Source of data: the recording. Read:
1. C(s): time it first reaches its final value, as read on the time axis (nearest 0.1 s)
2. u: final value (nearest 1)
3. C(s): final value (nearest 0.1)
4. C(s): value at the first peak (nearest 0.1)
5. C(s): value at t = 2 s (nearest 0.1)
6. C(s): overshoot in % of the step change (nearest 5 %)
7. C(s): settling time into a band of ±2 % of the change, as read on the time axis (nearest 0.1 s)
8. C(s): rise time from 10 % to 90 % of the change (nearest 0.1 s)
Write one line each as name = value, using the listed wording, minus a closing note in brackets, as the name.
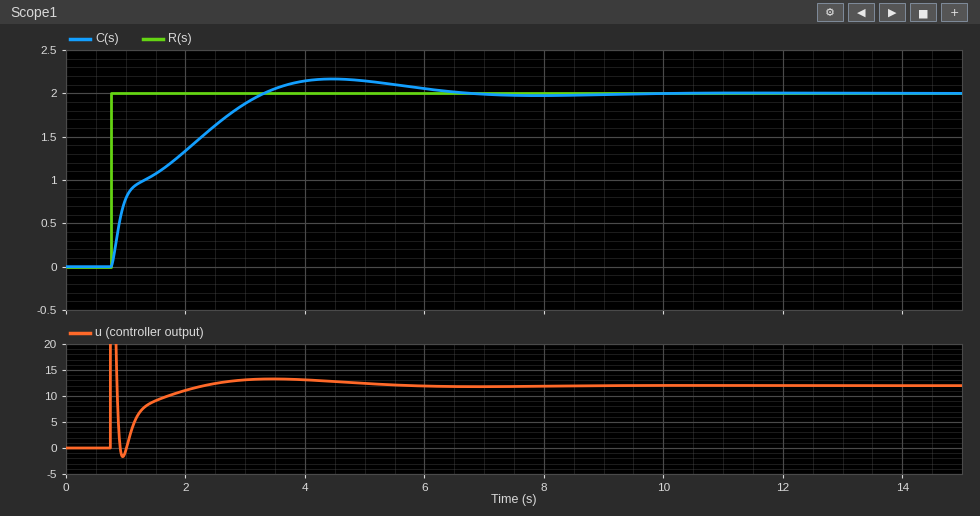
C(s): time it first reaches its final value, as read on the time axis = 3.3 s
u: final value = 12
C(s): final value = 2.0
C(s): value at the first peak = 2.2
C(s): value at t = 2 s = 1.3
C(s): overshoot in % of the step change = 10 %
C(s): settling time into a band of ±2 % of the change, as read on the time axis = 6.2 s
C(s): rise time from 10 % to 90 % of the change = 2.0 s
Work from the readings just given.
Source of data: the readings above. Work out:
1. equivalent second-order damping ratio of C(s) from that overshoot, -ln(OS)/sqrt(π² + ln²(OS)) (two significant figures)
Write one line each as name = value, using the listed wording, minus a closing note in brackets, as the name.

equivalent second-order damping ratio of C(s) from that overshoot, -ln(OS)/sqrt(π² + ln²(OS)) = 0.59
